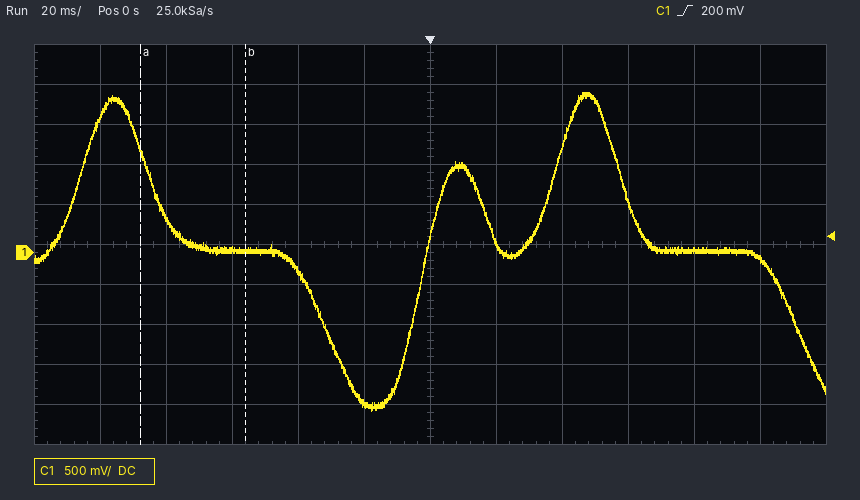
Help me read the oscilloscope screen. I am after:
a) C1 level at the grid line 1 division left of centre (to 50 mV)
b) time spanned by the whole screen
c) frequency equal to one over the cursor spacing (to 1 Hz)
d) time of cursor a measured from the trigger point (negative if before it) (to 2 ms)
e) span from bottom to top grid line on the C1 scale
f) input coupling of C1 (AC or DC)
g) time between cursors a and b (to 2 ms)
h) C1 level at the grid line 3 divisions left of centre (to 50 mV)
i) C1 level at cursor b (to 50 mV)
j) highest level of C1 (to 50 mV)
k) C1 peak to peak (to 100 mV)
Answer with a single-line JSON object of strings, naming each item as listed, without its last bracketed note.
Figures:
{"C1 level at the grid line 1 division left of centre": "-1.90 V", "time spanned by the whole screen": "240 ms", "frequency equal to one over the cursor spacing": "31 Hz", "time of cursor a measured from the trigger point (negative if before it)": "-88 ms", "span from bottom to top grid line on the C1 scale": "5 V", "input coupling of C1": "DC", "time between cursors a and b": "32 ms", "C1 level at the grid line 3 divisions left of centre": "50 mV", "C1 level at cursor b": "50 mV", "highest level of C1": "2.00 V", "C1 peak to peak": "4.00 V"}
